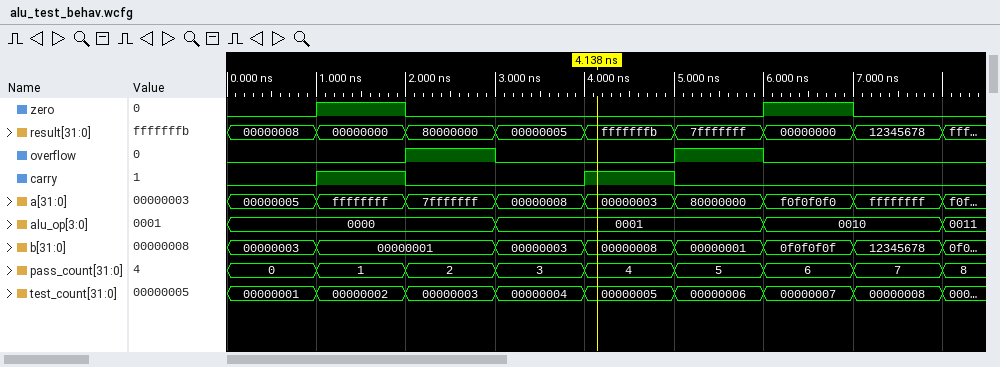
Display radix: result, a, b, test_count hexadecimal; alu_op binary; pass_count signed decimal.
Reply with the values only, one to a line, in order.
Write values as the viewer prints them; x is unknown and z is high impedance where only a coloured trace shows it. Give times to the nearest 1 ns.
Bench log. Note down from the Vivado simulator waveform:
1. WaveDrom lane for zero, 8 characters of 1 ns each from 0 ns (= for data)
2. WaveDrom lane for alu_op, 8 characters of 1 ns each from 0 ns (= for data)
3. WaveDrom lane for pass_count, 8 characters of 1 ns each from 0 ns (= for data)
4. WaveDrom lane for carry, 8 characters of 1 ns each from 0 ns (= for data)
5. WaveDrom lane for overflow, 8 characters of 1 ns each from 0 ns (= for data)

{name: 'zero', wave: '010...10'}
{name: 'alu_op', wave: '=..=..=.', data: '0000 0001 0010'}
{name: 'pass_count', wave: '========', data: '0 1 2 3 4 5 6 7'}
{name: 'carry', wave: '010.10..'}
{name: 'overflow', wave: '0.10.10.'}
